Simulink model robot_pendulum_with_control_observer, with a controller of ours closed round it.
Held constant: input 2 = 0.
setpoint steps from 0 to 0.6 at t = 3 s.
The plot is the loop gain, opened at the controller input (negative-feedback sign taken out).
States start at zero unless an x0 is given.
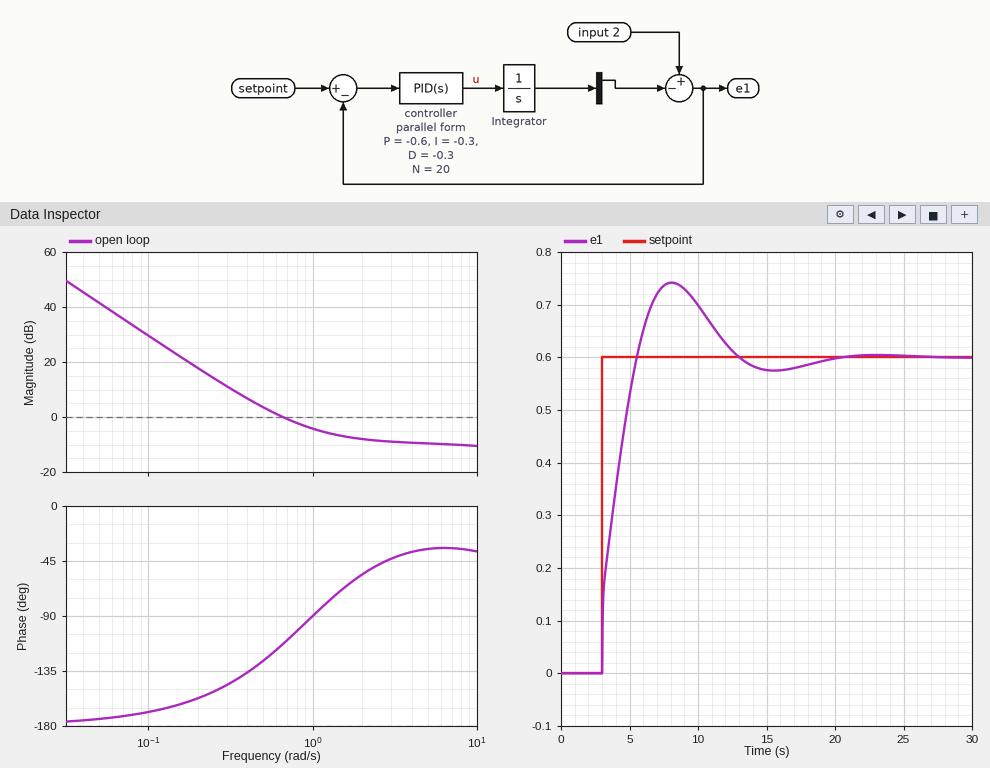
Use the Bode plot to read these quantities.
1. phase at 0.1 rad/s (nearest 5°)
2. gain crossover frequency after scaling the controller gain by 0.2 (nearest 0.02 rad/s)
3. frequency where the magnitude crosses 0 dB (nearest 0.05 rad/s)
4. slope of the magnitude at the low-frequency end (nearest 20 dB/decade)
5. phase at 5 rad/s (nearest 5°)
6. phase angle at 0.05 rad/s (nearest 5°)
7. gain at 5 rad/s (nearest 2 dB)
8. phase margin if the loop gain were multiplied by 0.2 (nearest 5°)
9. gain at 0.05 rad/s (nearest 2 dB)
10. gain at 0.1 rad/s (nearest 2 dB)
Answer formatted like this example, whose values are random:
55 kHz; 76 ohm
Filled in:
-170°; 0.26 rad/s; 0.65 rad/s; -40 dB/decade; -35°; -175°; -10 dB; 30°; 42 dB; 30 dB
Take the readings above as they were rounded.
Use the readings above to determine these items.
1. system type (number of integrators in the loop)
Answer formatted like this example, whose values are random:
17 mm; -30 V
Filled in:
2
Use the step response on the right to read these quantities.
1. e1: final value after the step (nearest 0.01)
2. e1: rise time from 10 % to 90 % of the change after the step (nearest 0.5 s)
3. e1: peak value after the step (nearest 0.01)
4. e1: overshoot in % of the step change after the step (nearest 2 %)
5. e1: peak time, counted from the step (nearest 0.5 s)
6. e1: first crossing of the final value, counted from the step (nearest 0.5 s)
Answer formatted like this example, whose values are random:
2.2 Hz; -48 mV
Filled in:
0.60; 2.0 s; 0.74; 24 %; 5.0 s; 2.5 s
